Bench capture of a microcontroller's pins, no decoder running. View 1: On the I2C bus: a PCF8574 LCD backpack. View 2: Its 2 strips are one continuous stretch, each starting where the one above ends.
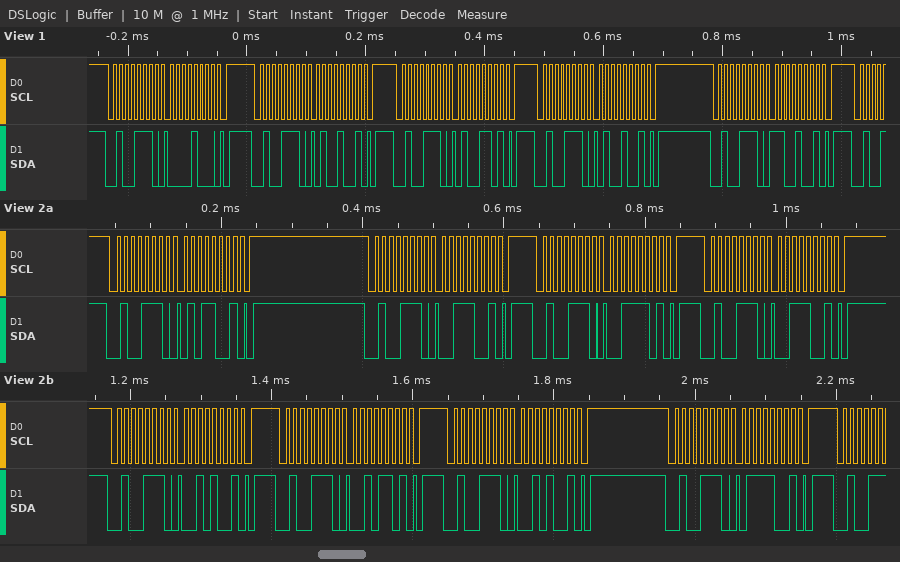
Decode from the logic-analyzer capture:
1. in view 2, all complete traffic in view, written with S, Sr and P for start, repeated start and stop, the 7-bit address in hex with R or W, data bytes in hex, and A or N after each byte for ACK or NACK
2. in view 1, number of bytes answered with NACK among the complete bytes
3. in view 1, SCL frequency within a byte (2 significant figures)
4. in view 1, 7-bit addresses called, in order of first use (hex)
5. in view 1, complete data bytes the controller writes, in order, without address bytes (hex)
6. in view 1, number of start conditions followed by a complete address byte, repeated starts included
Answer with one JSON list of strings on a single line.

["S 27W A 59 A P S 27W A 39 A P S 27W A 3D A P S 27W A 39 A P S 27W A 29 A P S 27W A 2D A P S 27W A 29 A P S 27W A 79 A P", "0", "100 kHz", "0x27", "08 49 4D 49 C9", "5"]
